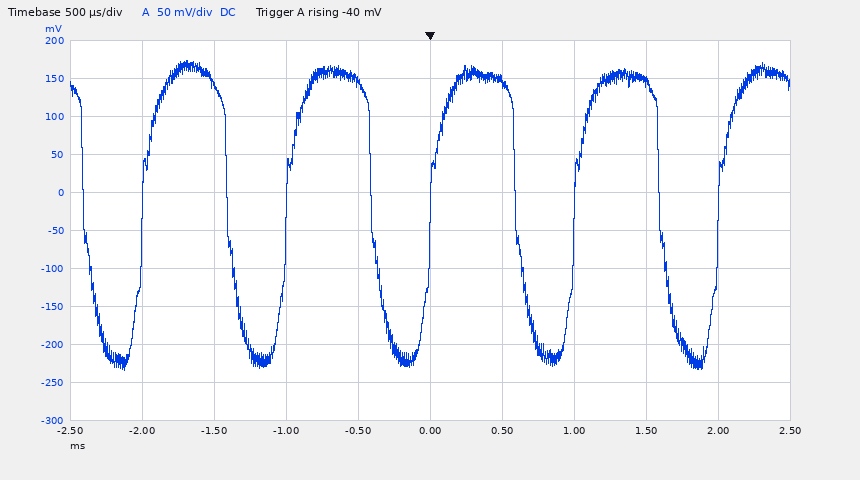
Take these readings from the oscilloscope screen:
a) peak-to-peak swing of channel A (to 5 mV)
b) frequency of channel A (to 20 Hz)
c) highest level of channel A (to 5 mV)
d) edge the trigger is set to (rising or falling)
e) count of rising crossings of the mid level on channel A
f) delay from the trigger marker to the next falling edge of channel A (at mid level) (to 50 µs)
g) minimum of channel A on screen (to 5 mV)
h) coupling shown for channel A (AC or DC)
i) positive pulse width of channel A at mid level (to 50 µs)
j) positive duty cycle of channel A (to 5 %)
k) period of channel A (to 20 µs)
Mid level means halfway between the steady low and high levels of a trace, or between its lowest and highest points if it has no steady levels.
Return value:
410 mV
1.00 kHz
175 mV
rising
5
600 µs
-235 mV
DC
600 µs
60 %
1.00 ms
